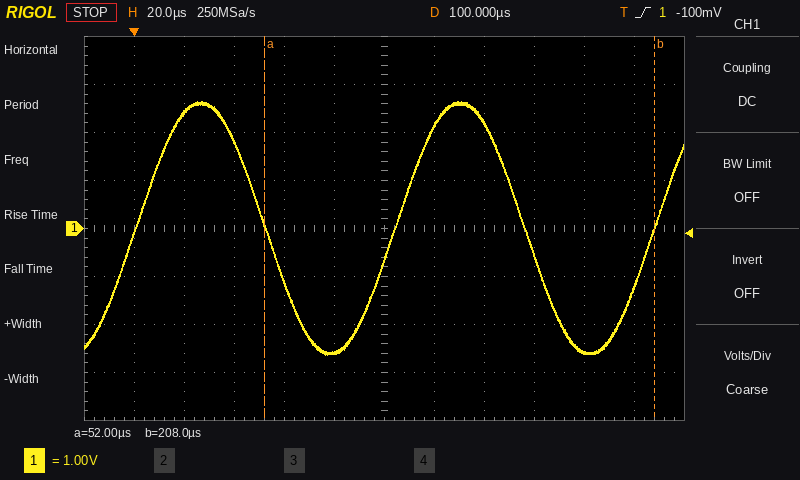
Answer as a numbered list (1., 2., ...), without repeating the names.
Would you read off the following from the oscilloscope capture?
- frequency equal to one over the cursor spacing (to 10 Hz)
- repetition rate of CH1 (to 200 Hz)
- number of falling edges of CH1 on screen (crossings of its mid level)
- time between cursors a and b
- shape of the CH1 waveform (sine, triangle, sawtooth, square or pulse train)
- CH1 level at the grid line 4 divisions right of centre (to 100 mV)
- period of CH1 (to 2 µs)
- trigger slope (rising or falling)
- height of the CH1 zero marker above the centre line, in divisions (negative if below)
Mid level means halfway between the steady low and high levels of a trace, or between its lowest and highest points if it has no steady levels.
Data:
1. 6.41 kHz
2. 9.6 kHz
3. 2
4. 156 µs
5. sine
6. -2.6 V
7. 104 µs
8. rising
9. 0.0 div
